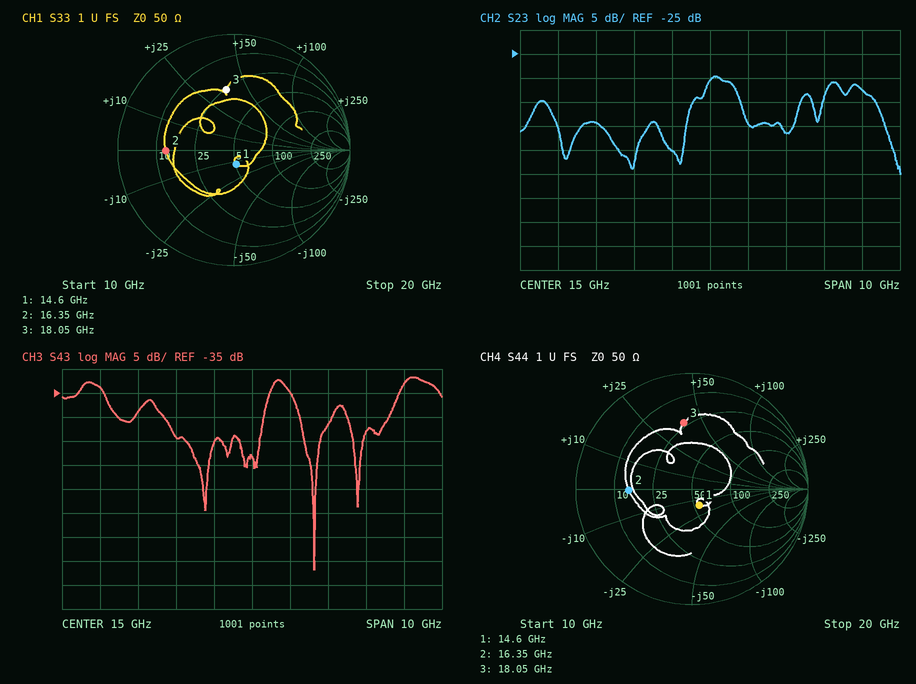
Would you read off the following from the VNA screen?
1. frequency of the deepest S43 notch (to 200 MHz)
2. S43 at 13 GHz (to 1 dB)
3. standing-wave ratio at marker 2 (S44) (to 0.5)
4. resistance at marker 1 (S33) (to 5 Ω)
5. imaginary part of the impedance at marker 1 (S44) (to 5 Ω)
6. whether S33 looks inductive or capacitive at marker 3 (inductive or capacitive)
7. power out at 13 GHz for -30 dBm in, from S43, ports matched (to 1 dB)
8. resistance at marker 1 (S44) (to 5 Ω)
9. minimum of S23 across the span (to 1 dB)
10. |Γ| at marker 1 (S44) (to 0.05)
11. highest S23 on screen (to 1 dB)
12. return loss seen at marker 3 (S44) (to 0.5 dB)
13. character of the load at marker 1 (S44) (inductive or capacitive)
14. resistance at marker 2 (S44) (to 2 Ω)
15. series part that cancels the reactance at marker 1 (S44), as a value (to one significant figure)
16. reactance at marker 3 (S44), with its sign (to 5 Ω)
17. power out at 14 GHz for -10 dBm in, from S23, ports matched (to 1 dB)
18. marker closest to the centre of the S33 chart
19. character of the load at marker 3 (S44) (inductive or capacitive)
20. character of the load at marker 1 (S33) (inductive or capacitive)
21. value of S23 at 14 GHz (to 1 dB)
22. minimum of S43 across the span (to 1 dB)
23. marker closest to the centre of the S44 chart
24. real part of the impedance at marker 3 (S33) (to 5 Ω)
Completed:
16.6 GHz
-44 dB
3.5
50 Ω
-15 Ω
inductive
-74 dBm
55 Ω
-50 dB
0.15
-30 dB
5.0 dB
capacitive
14 Ω
200 pH
+40 Ω
-55 dBm
marker 1
inductive
capacitive
-45 dB
-72 dB
marker 1
25 Ω
